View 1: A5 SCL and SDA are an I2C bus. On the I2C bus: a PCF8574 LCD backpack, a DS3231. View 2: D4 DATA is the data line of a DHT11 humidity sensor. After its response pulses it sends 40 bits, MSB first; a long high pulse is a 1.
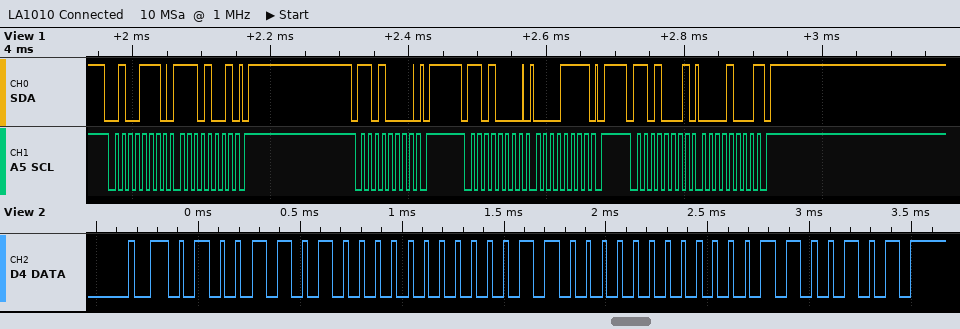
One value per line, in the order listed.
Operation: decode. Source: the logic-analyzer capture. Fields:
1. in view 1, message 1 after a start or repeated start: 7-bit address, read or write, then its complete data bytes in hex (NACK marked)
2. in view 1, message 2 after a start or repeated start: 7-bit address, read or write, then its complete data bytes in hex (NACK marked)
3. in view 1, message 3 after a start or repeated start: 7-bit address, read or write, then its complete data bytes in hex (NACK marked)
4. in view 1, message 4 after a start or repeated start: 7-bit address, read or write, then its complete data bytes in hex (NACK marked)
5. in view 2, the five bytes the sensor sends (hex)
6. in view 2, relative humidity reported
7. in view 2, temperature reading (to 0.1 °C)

0x27 write: E9
0x68 write
0x68 write: 0F
0x68 read: 08 NACK
4D 00 18 00 65
77 %
24.0 °C
